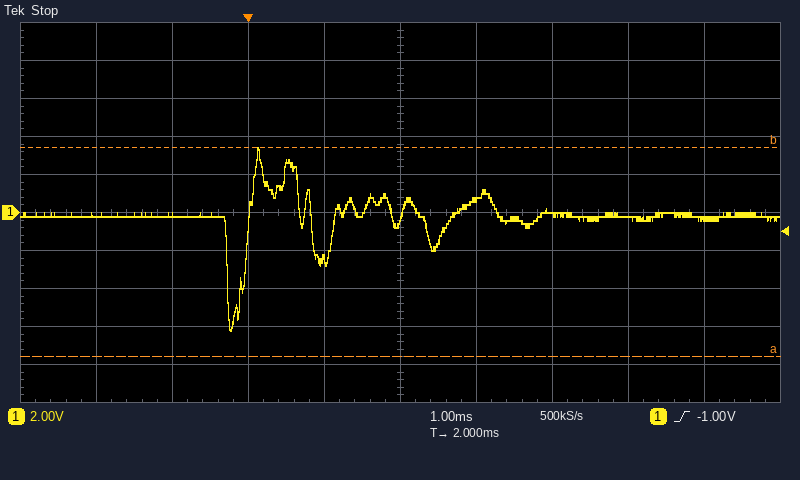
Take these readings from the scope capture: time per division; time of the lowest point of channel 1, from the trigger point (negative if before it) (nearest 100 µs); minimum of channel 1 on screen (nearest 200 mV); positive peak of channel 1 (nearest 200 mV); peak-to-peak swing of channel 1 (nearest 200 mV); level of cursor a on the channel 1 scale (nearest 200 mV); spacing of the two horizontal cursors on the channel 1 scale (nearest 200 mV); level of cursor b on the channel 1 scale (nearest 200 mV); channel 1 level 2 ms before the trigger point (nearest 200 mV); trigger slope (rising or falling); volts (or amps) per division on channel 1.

1 ms
-200 µs
-6.2 V
3.4 V
9.6 V
-7.6 V
11.0 V
3.4 V
-200 mV
rising
2 V
